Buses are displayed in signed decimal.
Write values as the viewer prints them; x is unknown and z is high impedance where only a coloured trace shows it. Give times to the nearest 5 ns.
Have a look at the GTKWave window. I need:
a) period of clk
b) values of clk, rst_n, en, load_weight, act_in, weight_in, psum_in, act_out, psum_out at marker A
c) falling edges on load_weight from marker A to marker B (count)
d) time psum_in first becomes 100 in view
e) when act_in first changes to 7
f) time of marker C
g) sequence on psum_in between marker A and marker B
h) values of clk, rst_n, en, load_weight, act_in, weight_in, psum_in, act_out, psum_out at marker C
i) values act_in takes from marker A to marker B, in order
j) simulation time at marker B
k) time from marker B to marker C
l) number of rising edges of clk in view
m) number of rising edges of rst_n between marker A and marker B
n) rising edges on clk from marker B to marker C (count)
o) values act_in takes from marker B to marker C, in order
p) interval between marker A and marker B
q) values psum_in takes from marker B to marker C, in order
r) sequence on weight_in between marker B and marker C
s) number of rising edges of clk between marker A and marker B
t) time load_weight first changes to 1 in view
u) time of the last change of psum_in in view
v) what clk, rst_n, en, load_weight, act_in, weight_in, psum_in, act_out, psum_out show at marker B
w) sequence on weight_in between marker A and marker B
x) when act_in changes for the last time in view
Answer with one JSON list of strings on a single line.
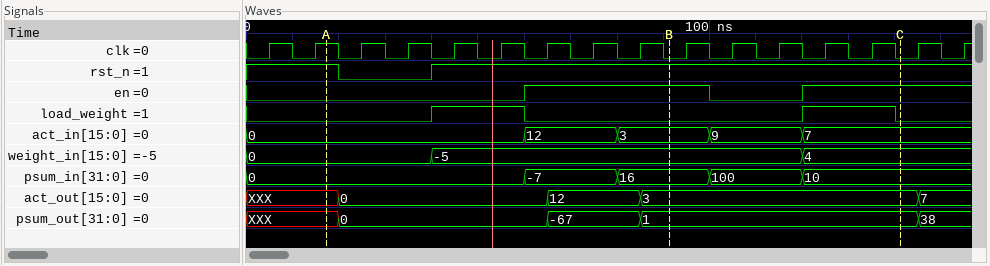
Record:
["10 ns", "clk=1, rst_n=1, en=0, load_weight=0, act_in=0, weight_in=0, psum_in=0, act_out=XXX, psum_out=XXX", "1", "100 ns", "120 ns", "140 ns", "0, -7, 16", "clk=0, rst_n=1, en=1, load_weight=0, act_in=7, weight_in=4, psum_in=10, act_out=3, psum_out=1", "0, 12, 3", "90 ns", "50 ns", "16", "1", "5", "3, 9, 7", "75 ns", "16, 100, 10", "-5, 4", "7", "40 ns", "120 ns", "clk=0, rst_n=1, en=1, load_weight=0, act_in=3, weight_in=-5, psum_in=16, act_out=3, psum_out=1", "0, -5", "120 ns"]
